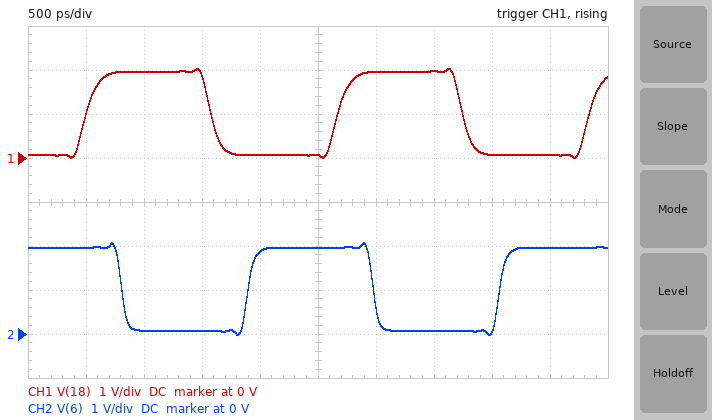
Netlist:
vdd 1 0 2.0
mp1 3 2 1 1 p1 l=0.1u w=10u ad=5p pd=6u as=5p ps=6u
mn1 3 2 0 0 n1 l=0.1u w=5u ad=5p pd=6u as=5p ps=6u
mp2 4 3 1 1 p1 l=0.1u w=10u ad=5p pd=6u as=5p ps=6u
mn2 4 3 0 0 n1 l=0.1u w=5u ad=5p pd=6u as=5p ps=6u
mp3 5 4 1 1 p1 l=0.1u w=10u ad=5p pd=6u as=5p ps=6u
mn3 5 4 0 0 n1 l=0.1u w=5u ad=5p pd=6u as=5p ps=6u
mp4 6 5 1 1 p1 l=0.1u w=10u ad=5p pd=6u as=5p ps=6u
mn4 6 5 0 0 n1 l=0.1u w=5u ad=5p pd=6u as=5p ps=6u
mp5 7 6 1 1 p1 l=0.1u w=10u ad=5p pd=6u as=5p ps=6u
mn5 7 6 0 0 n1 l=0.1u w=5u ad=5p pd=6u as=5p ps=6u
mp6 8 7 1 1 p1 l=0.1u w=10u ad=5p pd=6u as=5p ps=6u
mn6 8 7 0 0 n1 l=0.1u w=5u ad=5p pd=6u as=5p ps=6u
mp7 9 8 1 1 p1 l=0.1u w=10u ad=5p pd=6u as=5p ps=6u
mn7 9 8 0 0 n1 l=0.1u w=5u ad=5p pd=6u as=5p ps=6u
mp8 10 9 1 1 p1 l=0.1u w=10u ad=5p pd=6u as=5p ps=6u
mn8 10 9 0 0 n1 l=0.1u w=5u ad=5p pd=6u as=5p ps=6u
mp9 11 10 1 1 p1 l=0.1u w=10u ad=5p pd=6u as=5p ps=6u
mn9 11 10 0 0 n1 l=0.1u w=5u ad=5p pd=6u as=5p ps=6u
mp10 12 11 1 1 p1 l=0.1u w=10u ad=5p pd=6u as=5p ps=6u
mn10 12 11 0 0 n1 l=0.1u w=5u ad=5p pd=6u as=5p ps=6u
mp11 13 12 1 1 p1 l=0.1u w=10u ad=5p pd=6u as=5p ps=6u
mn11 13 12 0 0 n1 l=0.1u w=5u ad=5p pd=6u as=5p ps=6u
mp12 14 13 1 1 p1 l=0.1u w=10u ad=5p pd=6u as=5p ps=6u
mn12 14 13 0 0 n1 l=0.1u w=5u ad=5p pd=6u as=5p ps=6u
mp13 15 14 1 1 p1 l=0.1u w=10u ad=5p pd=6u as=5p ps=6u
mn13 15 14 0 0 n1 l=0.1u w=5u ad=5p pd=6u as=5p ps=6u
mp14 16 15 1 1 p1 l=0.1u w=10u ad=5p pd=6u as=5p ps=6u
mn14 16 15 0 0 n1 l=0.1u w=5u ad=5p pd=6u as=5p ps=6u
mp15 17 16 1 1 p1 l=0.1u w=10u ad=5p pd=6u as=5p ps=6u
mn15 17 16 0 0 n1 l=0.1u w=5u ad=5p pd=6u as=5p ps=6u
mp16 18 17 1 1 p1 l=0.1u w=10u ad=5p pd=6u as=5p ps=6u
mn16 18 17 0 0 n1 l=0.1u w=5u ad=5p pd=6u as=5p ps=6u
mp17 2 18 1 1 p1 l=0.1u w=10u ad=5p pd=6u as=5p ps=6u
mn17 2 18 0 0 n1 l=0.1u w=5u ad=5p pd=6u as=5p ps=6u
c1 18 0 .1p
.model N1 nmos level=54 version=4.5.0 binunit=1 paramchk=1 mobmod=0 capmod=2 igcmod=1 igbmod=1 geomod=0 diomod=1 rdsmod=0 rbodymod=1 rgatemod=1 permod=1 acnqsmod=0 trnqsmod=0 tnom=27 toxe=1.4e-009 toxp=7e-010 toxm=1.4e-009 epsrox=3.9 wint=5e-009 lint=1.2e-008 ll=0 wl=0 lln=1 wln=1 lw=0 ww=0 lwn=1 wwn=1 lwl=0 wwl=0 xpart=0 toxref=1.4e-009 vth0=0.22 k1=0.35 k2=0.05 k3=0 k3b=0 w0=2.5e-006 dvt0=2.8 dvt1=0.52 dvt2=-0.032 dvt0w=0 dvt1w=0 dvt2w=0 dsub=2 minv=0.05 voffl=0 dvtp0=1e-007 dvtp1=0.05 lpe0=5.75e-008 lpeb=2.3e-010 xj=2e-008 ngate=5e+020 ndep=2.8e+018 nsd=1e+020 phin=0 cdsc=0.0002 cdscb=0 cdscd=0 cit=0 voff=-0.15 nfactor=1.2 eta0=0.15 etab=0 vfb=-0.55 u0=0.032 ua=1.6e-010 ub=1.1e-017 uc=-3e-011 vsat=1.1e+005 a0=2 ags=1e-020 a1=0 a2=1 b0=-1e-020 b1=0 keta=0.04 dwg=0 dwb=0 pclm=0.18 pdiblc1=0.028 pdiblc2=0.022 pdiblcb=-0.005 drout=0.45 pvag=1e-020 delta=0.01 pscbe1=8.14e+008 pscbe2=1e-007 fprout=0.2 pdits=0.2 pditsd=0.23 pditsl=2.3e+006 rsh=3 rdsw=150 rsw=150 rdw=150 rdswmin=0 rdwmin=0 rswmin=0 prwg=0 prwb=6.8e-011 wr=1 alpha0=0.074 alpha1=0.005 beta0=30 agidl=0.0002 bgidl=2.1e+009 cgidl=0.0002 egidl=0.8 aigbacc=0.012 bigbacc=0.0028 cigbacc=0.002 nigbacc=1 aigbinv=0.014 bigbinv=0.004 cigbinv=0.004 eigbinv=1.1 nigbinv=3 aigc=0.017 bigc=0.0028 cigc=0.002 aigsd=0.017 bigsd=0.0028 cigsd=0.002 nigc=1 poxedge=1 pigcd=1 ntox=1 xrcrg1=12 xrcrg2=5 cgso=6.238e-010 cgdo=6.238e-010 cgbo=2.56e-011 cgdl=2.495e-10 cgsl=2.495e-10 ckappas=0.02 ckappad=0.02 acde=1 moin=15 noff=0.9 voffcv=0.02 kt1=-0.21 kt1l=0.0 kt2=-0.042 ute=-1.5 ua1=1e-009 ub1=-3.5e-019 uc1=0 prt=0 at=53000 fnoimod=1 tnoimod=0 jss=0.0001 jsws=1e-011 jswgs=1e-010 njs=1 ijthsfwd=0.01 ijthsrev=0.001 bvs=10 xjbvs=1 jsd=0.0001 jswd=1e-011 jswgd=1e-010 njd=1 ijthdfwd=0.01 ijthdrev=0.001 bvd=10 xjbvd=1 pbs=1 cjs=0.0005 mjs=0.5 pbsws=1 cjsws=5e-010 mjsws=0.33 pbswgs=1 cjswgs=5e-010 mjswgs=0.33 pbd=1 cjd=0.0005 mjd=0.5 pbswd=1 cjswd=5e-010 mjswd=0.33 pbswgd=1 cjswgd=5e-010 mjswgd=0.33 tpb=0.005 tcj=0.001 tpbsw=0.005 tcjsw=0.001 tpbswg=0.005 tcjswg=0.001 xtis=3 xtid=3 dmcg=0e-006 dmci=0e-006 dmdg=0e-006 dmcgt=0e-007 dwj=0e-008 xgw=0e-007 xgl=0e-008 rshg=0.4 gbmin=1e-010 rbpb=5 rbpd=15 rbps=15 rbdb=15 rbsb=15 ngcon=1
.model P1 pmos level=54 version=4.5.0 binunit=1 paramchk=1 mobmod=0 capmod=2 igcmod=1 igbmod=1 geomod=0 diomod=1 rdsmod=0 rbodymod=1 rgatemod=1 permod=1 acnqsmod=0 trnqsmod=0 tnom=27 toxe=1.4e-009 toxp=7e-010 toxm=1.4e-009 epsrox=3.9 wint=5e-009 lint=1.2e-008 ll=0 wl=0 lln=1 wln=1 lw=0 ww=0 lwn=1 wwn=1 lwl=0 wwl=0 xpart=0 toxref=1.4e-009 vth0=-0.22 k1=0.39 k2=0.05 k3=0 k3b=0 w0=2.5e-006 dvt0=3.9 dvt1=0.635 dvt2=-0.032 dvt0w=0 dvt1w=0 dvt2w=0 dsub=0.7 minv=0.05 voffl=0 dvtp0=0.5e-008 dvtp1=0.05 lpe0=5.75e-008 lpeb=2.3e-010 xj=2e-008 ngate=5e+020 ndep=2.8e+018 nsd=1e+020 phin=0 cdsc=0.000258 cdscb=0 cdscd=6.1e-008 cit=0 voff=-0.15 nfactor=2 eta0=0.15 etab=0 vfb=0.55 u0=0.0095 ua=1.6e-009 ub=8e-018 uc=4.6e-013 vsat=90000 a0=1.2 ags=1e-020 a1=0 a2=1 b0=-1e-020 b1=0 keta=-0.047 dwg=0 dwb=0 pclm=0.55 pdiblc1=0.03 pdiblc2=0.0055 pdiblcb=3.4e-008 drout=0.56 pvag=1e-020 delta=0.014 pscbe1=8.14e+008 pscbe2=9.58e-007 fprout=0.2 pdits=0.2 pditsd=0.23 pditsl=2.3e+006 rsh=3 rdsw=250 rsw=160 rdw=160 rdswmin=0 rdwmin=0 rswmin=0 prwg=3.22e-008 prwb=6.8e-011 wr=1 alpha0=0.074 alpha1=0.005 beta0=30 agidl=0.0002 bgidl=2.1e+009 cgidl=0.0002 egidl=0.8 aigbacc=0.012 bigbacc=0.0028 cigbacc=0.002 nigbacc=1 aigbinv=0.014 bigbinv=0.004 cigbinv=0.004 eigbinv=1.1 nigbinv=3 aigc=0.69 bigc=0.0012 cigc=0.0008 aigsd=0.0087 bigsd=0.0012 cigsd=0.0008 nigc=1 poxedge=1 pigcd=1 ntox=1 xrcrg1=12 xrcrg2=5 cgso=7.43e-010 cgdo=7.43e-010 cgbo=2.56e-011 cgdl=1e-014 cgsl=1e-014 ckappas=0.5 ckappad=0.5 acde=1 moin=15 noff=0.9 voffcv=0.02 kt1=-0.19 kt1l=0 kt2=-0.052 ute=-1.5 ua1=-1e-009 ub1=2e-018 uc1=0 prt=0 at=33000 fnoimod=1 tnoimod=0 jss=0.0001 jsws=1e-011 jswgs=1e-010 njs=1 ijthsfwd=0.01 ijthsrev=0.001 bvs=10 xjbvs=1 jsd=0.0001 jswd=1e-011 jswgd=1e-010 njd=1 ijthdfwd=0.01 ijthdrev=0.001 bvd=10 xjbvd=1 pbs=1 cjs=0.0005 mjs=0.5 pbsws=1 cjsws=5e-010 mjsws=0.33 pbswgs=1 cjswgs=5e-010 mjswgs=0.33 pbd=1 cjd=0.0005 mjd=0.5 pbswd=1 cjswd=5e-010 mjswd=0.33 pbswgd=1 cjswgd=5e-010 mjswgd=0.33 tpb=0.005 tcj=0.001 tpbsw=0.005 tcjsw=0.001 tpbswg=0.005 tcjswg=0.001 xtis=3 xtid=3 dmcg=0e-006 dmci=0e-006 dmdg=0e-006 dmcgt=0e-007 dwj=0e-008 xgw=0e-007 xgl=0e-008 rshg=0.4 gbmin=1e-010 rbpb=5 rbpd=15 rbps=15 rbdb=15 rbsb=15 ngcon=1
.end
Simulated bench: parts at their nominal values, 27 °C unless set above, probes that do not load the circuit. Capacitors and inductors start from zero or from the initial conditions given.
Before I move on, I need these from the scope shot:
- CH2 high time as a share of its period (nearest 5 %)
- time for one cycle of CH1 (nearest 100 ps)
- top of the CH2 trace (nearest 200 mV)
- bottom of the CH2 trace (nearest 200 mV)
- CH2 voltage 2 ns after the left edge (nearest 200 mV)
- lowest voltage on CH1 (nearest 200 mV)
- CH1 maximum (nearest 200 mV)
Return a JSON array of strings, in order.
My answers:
["50 %", "2.2 ns", "2.0 V", "0 V", "1.8 V", "0 V", "2.0 V"]
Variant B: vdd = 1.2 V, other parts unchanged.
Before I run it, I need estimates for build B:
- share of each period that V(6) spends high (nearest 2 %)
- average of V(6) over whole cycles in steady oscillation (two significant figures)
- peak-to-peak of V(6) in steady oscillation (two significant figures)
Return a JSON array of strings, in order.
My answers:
["50 %", "600 mV", "1.3 V"]
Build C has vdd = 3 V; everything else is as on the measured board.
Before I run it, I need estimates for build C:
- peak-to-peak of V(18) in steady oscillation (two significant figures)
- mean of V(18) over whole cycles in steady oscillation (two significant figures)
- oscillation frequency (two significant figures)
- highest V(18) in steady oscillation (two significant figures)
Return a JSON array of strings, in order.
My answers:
["1.7 V", "1.5 V", "480 MHz", "2.4 V"]
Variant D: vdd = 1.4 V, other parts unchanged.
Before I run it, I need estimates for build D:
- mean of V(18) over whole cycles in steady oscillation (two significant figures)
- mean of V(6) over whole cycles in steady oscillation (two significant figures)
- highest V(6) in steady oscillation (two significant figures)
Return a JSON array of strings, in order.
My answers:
["690 mV", "700 mV", "1.5 V"]
